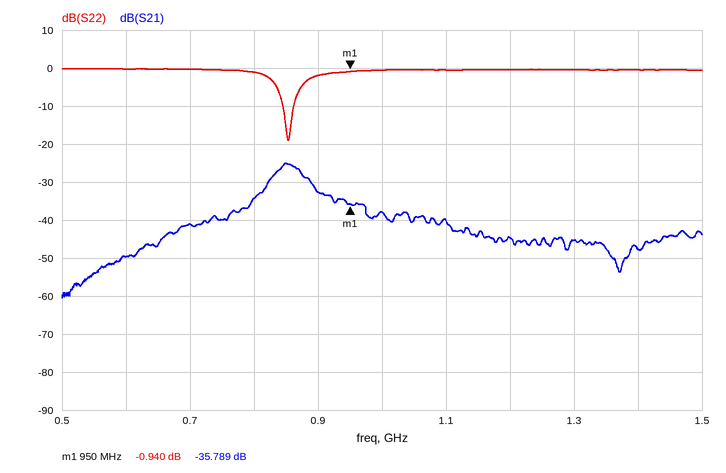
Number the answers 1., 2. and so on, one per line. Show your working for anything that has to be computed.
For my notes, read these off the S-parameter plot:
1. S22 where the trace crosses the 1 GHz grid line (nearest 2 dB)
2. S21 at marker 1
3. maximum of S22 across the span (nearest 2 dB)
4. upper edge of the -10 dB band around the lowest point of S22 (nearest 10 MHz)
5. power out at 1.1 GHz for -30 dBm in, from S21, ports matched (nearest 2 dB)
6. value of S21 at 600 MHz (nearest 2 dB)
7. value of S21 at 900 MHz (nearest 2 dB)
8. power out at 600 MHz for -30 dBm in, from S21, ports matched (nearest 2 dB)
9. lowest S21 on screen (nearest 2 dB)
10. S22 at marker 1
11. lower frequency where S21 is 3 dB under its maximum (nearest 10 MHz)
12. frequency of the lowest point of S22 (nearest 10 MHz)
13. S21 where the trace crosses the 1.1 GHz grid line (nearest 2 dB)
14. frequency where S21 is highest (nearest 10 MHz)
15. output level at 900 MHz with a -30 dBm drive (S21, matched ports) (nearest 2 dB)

1. 0 dB
2. -35.789 dB
3. 0 dB
4. 860 MHz
5. -30 dBm + (-40 dB) = -70 dBm
6. -50 dB
7. -32 dB
8. -30 dBm + (-50 dB) = -80 dBm
9. -60 dB
10. -0.940 dB
11. 830 MHz
12. 850 MHz
13. -40 dB
14. 850 MHz
15. -30 dBm + (-32 dB) = -62 dBm
